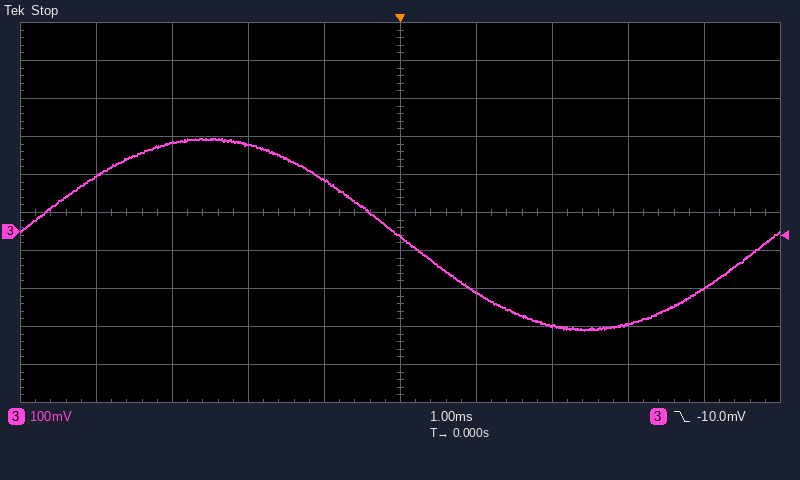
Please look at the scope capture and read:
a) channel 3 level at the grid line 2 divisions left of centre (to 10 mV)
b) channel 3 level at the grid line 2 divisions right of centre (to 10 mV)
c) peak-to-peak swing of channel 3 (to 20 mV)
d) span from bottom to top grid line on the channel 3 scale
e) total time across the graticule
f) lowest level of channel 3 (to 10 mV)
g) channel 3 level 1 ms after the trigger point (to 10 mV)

230 mV
-250 mV
500 mV
1 V
10 ms
-260 mV
-160 mV
